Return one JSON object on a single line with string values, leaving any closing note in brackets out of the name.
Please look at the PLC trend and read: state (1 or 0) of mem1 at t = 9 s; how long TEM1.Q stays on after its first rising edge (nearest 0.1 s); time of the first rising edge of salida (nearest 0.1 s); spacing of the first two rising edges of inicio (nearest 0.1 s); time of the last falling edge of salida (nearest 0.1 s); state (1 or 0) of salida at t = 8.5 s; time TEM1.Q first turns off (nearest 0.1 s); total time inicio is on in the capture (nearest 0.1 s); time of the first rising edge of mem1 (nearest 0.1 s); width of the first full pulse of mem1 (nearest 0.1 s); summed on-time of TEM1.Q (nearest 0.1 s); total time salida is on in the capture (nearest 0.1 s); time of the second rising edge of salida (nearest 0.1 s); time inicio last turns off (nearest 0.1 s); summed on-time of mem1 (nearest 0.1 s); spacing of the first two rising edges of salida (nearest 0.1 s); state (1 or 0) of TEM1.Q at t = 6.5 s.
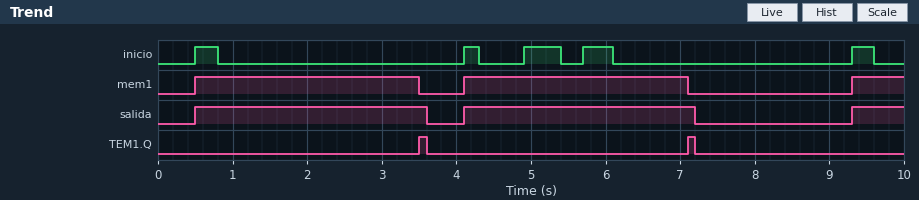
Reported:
{"state (1 or 0) of mem1 at t = 9 s": "0", "how long TEM1.Q stays on after its first rising edge": "0.1 s", "time of the first rising edge of salida": "0.5 s", "spacing of the first two rising edges of inicio": "3.6 s", "time of the last falling edge of salida": "7.2 s", "state (1 or 0) of salida at t = 8.5 s": "0", "time TEM1.Q first turns off": "3.6 s", "total time inicio is on in the capture": "1.7 s", "time of the first rising edge of mem1": "0.5 s", "width of the first full pulse of mem1": "3.0 s", "summed on-time of TEM1.Q": "0.2 s", "total time salida is on in the capture": "6.9 s", "time of the second rising edge of salida": "4.1 s", "time inicio last turns off": "9.6 s", "summed on-time of mem1": "6.7 s", "spacing of the first two rising edges of salida": "3.6 s", "state (1 or 0) of TEM1.Q at t = 6.5 s": "0"}
